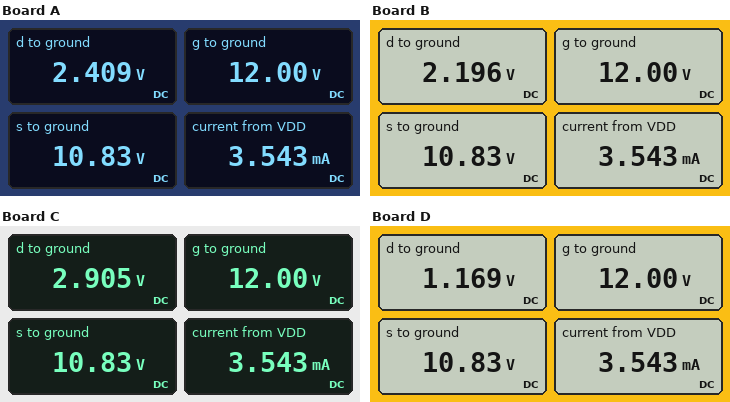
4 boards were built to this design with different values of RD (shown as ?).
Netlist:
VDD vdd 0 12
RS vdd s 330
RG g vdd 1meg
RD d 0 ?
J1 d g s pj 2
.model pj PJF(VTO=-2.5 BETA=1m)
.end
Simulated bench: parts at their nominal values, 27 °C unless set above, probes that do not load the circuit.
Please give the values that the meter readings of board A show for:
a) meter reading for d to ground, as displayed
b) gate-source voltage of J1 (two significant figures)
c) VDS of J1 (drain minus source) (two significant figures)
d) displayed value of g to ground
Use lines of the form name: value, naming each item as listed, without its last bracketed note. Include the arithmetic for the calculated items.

meter reading for d to ground, as displayed: 2.409 V
gate-source voltage of J1: 12 V - 10.83 V = 1.2 V
VDS of J1 (drain minus source): 2.409 V - 10.83 V = -8.4 V
displayed value of g to ground: 12.00 V
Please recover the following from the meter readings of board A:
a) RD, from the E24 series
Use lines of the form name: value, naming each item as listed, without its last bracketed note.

RD, from the E24 series: 680 Ω
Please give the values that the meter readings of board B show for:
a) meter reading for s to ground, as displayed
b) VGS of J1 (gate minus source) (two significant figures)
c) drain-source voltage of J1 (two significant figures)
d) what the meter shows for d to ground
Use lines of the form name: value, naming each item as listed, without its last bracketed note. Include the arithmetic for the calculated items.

meter reading for s to ground, as displayed: 10.83 V
VGS of J1 (gate minus source): 12 V - 10.83 V = 1.2 V
drain-source voltage of J1: 2.196 V - 10.83 V = -8.6 V
what the meter shows for d to ground: 2.196 V
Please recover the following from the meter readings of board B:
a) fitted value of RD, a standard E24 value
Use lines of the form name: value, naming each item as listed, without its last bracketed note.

fitted value of RD, a standard E24 value: 620 Ω
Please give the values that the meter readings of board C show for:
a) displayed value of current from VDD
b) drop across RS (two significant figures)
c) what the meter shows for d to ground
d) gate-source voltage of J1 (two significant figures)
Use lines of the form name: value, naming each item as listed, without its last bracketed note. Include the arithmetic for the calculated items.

displayed value of current from VDD: 3.543 mA
drop across RS: 12 V - 10.83 V = 1.2 V
what the meter shows for d to ground: 2.905 V
gate-source voltage of J1: 12 V - 10.83 V = 1.2 V
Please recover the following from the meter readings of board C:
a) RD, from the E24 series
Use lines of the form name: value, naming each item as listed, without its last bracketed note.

RD, from the E24 series: 820 Ω
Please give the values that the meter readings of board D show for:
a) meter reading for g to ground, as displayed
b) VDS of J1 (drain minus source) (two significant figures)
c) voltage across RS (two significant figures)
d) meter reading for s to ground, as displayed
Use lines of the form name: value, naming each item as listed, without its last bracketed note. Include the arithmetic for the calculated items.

meter reading for g to ground, as displayed: 12.00 V
VDS of J1 (drain minus source): 1.169 V - 10.83 V = -9.7 V
voltage across RS: 12 V - 10.83 V = 1.2 V
meter reading for s to ground, as displayed: 10.83 V
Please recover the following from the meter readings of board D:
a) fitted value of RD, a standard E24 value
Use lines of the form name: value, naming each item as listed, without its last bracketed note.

fitted value of RD, a standard E24 value: 330 Ω
